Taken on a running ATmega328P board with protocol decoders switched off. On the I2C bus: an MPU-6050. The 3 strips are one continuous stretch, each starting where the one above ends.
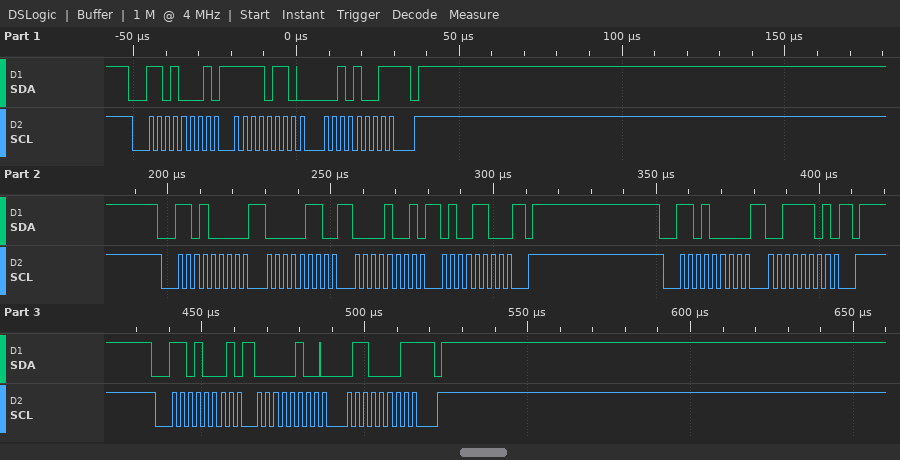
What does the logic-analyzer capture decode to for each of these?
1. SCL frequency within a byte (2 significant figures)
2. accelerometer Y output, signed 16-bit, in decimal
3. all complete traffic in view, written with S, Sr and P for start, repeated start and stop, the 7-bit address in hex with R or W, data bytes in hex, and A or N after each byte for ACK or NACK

400 kHz
1121
S 68R A F6 A 29 N P S 68W A 06 A 09 A 4C A P S 68W A 3D A P S 68R A 04 A 61 N P
